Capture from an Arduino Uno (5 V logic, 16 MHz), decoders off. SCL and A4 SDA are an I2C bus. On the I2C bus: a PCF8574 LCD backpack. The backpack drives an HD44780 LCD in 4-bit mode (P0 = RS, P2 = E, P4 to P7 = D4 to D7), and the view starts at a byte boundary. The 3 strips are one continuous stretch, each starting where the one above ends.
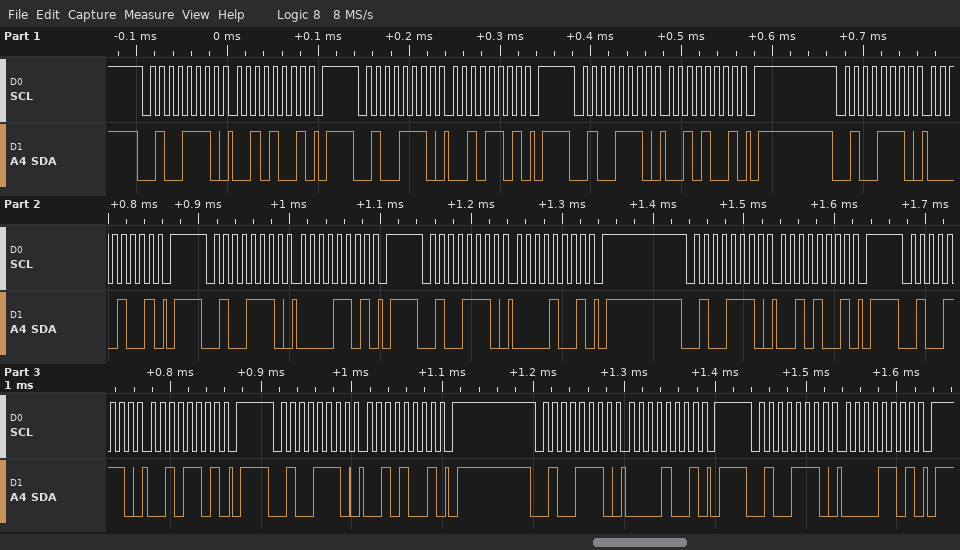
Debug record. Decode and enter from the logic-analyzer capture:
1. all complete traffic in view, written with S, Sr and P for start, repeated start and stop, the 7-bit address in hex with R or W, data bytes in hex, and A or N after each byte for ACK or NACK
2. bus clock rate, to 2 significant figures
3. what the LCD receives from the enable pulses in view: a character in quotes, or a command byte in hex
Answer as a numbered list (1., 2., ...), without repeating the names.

1. S 27W A 29 A P S 27W A 2D A P S 27W A 29 A P S 27W A 09 A P S 27W A 0D A P S 27W A 09 A P S 27W A 29 A P S 27W A 2D A P S 27W A 29 A P S 27W A 09 A P S 27W A 0D A P
2. 100 kHz
3. ' '
